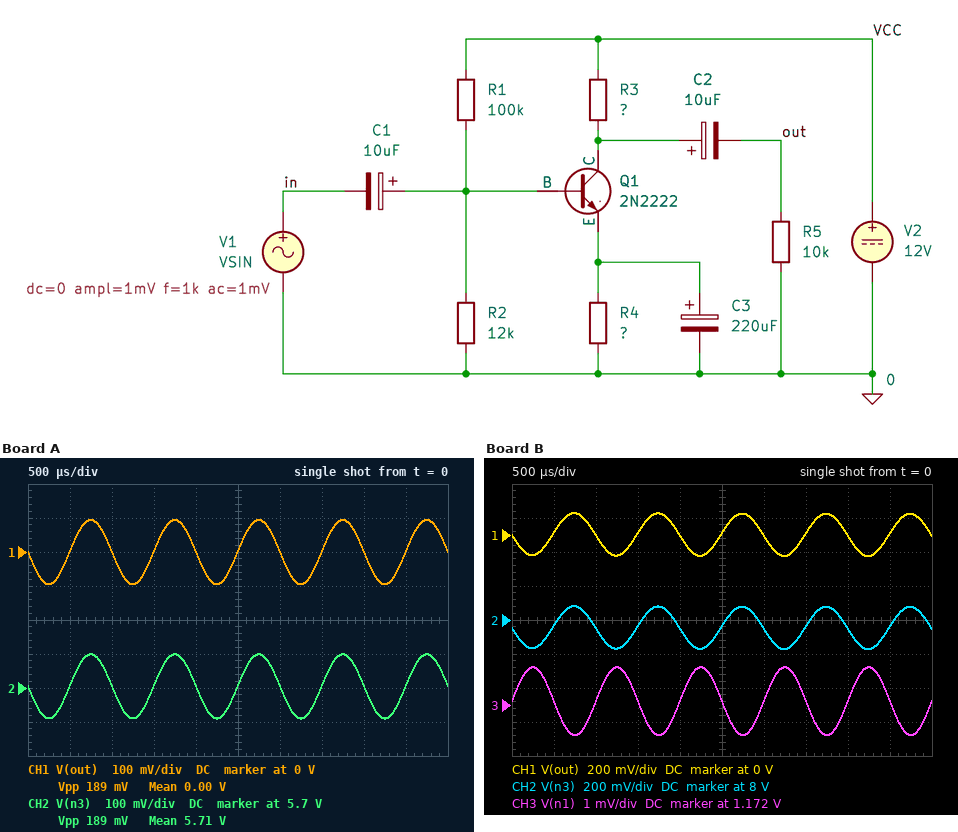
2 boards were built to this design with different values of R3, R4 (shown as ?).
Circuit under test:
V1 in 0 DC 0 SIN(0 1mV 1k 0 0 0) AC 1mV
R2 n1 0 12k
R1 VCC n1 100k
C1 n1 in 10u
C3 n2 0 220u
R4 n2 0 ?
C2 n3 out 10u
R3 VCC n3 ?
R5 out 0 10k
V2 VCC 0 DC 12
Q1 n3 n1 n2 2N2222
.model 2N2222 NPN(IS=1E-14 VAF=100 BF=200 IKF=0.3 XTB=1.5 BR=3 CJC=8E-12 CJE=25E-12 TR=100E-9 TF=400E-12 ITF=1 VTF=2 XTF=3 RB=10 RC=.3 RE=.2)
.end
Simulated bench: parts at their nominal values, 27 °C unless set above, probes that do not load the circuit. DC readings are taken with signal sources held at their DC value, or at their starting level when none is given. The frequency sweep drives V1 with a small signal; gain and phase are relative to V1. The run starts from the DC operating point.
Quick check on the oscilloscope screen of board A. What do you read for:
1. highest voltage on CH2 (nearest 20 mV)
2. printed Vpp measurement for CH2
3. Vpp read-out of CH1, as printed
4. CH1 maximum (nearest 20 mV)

5.80 V
189 mV
189 mV
100 mV
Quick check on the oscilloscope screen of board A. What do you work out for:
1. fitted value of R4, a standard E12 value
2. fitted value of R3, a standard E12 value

1.5 kΩ
15 kΩ
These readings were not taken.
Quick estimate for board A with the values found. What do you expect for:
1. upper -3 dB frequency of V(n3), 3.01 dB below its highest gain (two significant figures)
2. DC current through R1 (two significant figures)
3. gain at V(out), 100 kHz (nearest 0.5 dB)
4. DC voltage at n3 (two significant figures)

5.5 MHz
110 µA
39.5 dB
5.7 V
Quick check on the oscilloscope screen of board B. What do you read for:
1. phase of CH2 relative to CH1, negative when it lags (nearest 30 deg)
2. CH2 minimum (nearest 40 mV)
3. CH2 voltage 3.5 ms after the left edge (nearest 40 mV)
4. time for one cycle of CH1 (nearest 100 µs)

0 deg
7.84 V
7.96 V
1.0 ms
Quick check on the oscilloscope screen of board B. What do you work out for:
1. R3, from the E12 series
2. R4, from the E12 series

1.8 kΩ
220 Ω
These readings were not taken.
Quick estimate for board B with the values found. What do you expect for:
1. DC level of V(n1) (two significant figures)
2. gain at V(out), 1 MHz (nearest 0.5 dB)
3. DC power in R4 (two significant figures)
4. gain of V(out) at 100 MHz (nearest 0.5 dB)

1.2 V
42.0 dB
1.1 mW
25.0 dB
